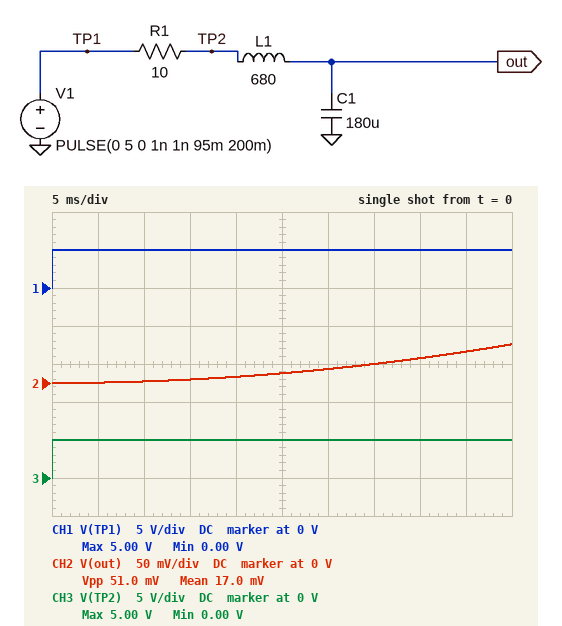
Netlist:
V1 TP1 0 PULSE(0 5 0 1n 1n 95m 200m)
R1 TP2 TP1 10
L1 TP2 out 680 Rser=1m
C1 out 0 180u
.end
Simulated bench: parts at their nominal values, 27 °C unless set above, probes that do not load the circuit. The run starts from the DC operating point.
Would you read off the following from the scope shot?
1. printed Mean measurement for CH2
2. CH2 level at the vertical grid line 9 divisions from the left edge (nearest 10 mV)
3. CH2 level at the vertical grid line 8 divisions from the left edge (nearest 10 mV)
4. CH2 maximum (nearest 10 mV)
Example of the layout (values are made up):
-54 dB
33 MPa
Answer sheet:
17.0 mV
40 mV
30 mV
50 mV
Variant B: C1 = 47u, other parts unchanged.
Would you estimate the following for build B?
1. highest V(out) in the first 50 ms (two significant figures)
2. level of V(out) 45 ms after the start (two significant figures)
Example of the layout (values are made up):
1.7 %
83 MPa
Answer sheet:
190 mV
160 mV
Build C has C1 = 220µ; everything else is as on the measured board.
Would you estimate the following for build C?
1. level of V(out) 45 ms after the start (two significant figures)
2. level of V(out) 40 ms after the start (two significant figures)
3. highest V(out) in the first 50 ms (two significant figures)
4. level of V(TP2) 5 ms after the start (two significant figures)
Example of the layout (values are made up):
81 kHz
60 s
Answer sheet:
34 mV
27 mV
42 mV
5.0 V
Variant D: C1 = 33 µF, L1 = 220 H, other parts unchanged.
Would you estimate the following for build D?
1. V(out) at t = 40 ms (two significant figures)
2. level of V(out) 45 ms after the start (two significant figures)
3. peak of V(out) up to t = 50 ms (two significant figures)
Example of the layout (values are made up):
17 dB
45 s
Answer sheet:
540 mV
680 mV
840 mV
